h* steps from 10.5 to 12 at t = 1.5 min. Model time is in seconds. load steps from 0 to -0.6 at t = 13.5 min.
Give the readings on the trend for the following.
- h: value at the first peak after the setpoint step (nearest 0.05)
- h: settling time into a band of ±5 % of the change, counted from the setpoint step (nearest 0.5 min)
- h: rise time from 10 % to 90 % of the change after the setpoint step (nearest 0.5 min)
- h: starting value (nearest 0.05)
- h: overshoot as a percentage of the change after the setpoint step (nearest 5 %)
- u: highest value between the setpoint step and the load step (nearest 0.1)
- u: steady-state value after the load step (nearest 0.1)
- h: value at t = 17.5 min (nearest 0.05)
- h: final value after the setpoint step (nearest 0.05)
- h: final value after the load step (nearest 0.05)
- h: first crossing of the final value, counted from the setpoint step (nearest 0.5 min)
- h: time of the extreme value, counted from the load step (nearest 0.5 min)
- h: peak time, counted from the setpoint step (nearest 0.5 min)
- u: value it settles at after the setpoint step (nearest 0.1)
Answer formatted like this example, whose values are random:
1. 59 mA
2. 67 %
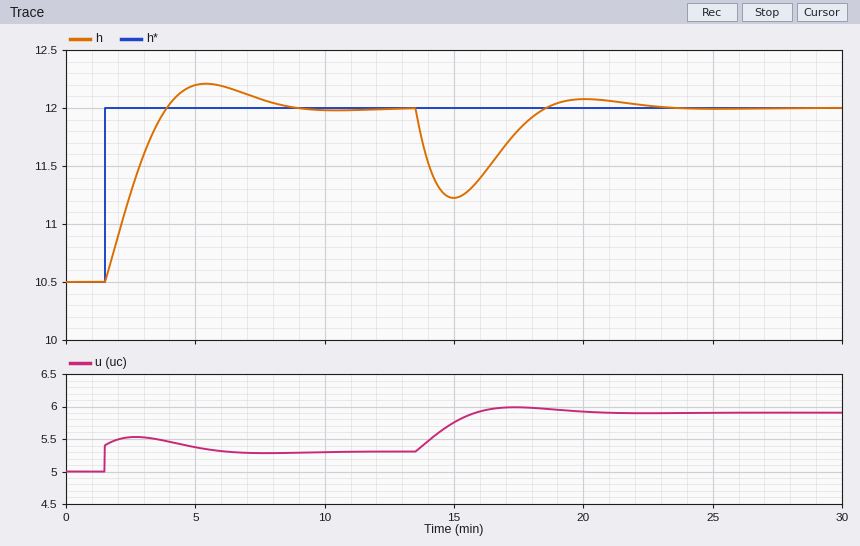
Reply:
1. 12.20
2. 6.0 min
3. 2.0 min
4. 10.50
5. 15 %
6. 5.5
7. 5.9
8. 11.80
9. 12.00
10. 12.00
11. 2.5 min
12. 1.5 min
13. 4.0 min
14. 5.3
